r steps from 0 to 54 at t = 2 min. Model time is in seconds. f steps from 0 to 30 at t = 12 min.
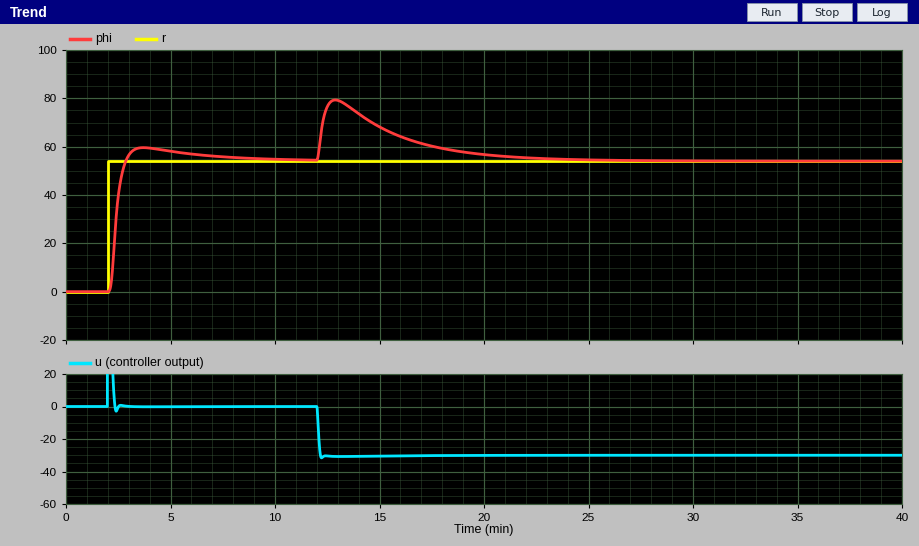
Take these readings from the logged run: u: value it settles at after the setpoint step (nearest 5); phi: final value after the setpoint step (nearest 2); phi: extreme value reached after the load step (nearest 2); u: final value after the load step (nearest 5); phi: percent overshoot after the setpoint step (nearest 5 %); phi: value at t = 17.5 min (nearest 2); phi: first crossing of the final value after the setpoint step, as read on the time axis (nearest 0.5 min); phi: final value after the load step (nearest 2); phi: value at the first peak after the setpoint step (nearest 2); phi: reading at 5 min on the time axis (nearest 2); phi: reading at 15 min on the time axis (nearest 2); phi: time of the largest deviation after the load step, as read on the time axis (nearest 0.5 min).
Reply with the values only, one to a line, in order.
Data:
0
54
80
-30
10 %
60
3.0 min
54
60
58
68
13.0 min
